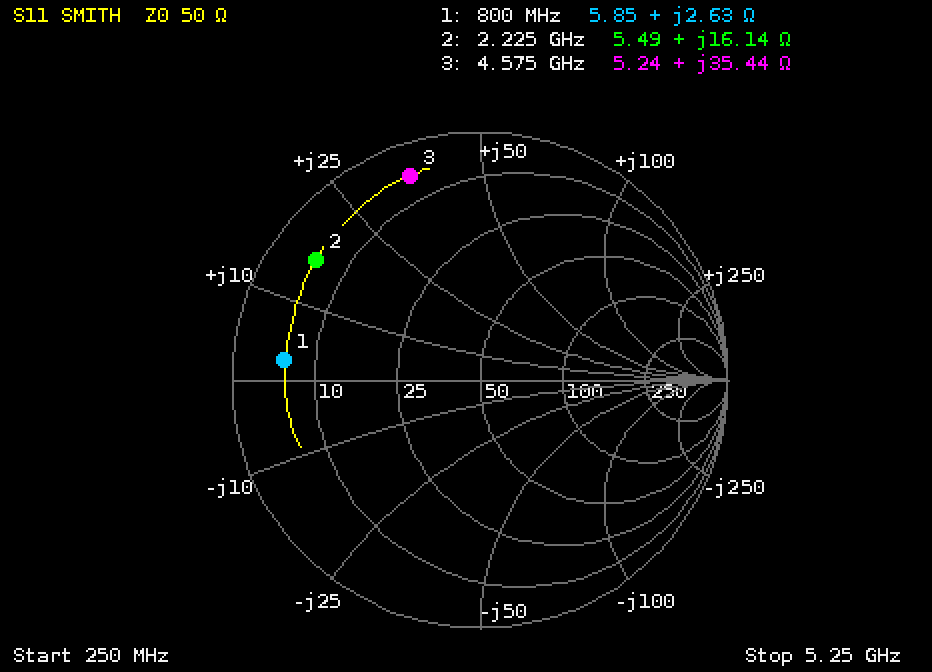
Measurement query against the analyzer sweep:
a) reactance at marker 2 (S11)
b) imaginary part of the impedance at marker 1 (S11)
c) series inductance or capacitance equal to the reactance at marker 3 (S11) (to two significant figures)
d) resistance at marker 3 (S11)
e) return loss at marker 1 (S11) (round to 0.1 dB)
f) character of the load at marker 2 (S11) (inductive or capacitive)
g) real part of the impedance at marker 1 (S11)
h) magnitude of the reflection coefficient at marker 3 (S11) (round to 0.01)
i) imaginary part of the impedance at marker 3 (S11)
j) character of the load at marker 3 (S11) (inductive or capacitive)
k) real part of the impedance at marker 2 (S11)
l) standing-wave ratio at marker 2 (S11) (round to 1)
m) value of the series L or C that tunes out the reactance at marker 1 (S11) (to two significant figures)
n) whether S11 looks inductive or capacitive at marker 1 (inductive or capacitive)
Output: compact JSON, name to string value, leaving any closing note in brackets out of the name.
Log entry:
{"reactance at marker 2": "+16.14 Ω", "imaginary part of the impedance at marker 1": "+2.63 Ω", "series inductance or capacitance equal to the reactance at marker 3 (S11)": "1.2 nH", "resistance at marker 3": "5.24 Ω", "return loss at marker 1 (S11)": "2.0 dB", "character of the load at marker 2 (S11)": "inductive", "real part of the impedance at marker 1": "5.85 Ω", "magnitude of the reflection coefficient at marker 3 (S11)": "0.87", "imaginary part of the impedance at marker 3": "+35.44 Ω", "character of the load at marker 3 (S11)": "inductive", "real part of the impedance at marker 2": "5.49 Ω", "standing-wave ratio at marker 2 (S11)": "10", "value of the series L or C that tunes out the reactance at marker 1 (S11)": "76 pF", "whether S11 looks inductive or capacitive at marker 1": "inductive"}
